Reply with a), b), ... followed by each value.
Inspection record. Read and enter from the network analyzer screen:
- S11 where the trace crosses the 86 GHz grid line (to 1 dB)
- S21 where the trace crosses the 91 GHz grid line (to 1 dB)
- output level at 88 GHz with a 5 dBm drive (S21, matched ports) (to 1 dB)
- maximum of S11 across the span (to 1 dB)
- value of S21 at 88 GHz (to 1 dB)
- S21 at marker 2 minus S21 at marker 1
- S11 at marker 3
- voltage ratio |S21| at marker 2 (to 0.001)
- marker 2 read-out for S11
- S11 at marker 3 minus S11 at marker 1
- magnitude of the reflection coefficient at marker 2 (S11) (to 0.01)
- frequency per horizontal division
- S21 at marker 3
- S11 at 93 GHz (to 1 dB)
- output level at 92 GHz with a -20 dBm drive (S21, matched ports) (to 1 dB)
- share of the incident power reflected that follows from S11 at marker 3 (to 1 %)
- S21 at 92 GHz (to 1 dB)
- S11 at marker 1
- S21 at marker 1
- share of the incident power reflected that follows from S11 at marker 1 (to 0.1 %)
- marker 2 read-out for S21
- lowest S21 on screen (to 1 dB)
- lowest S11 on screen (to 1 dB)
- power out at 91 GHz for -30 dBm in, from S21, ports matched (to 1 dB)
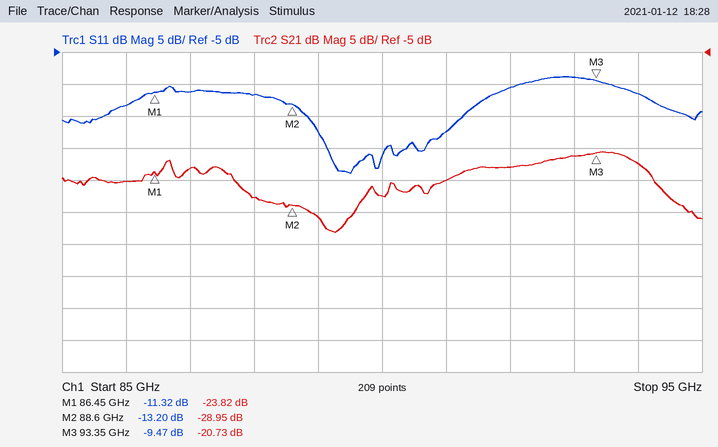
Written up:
a) -13 dB
b) -25 dB
c) -23 dBm
d) -9 dB
e) -28 dB
f) -5.13 dB
g) -9.47 dB
h) 0.036
i) -13.20 dB
j) 1.85 dB
k) 0.22
l) 1 GHz
m) -20.73 dB
n) -9 dB
o) -43 dBm
p) 11 %
q) -23 dB
r) -11.32 dB
s) -23.82 dB
t) 7.4 %
u) -28.95 dB
v) -33 dB
w) -24 dB
x) -55 dBm
